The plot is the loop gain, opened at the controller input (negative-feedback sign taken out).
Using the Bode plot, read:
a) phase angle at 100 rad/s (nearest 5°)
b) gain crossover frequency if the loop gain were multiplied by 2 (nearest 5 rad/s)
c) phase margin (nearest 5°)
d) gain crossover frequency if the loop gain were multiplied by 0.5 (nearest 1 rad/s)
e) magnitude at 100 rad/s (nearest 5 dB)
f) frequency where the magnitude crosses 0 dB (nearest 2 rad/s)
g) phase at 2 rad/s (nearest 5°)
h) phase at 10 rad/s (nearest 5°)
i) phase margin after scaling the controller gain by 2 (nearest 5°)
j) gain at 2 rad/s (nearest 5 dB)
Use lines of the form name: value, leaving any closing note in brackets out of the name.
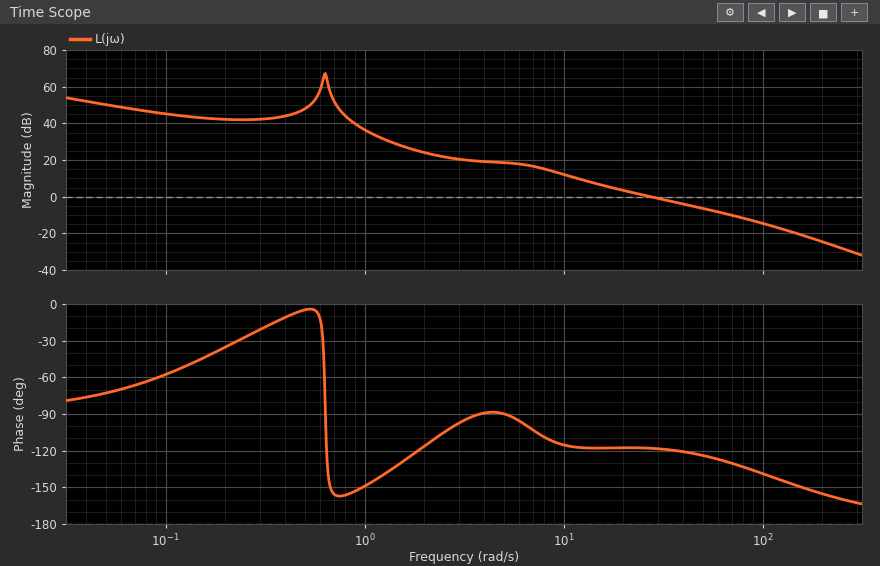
phase angle at 100 rad/s: -140°
gain crossover frequency if the loop gain were multiplied by 2: 50 rad/s
phase margin: 60°
gain crossover frequency if the loop gain were multiplied by 0.5: 16 rad/s
magnitude at 100 rad/s: -15 dB
frequency where the magnitude crosses 0 dB: 28 rad/s
phase at 2 rad/s: -115°
phase at 10 rad/s: -115°
phase margin after scaling the controller gain by 2: 55°
gain at 2 rad/s: 25 dB
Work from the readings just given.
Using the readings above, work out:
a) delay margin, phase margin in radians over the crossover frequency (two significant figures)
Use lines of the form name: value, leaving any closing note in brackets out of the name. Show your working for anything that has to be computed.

delay margin, phase margin in radians over the crossover frequency: 60 × π / 180 / 28 = 0.037 s
